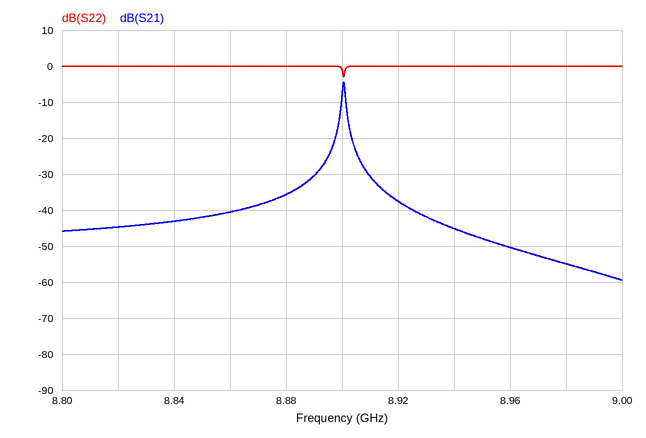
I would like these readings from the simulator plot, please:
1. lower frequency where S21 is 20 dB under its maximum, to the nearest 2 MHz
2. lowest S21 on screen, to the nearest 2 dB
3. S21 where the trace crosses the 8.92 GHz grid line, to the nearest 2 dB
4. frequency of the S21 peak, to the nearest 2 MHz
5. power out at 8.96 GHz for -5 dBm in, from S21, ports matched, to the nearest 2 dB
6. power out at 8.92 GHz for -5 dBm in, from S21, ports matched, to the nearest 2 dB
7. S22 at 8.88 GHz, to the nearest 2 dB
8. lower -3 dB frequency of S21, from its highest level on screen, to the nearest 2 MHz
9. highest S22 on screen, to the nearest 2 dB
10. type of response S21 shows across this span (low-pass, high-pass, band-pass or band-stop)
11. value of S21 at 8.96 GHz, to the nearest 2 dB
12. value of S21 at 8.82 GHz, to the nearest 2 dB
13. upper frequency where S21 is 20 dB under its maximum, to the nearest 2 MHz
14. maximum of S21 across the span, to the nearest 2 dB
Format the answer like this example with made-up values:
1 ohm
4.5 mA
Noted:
8.896 GHz
-60 dB
-38 dB
8.900 GHz
-56 dBm
-42 dBm
0 dB
8.900 GHz
0 dB
band-pass
-50 dB
-44 dB
8.906 GHz
-4 dB
